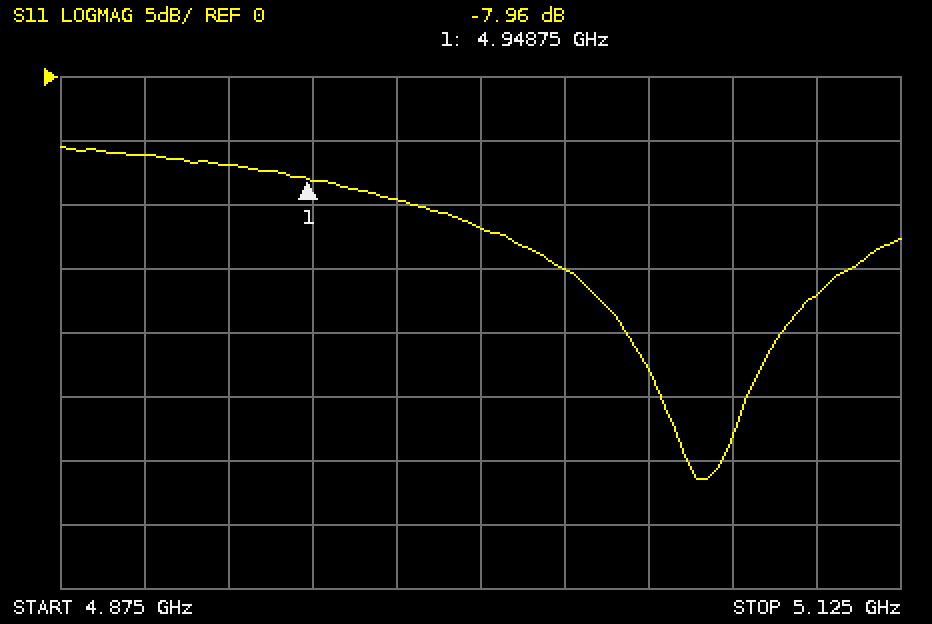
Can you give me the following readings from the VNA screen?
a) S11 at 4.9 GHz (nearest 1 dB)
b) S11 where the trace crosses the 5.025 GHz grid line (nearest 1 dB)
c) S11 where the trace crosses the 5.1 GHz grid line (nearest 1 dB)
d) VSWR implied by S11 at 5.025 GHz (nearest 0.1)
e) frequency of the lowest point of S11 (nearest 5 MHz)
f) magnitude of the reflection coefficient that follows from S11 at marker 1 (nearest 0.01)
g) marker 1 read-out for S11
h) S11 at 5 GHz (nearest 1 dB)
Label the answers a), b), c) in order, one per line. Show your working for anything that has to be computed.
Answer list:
a) -6 dB
b) -15 dB
c) -17 dB
d) |Γ| = 10^(-15/20) = 0.1778; VSWR = (1 + 0.1778)/(1 − 0.1778) ≈ 1.4
e) 5.065 GHz
f) 10^(-7.96/20) ≈ 0.40
g) -7.96 dB
h) -12 dB
